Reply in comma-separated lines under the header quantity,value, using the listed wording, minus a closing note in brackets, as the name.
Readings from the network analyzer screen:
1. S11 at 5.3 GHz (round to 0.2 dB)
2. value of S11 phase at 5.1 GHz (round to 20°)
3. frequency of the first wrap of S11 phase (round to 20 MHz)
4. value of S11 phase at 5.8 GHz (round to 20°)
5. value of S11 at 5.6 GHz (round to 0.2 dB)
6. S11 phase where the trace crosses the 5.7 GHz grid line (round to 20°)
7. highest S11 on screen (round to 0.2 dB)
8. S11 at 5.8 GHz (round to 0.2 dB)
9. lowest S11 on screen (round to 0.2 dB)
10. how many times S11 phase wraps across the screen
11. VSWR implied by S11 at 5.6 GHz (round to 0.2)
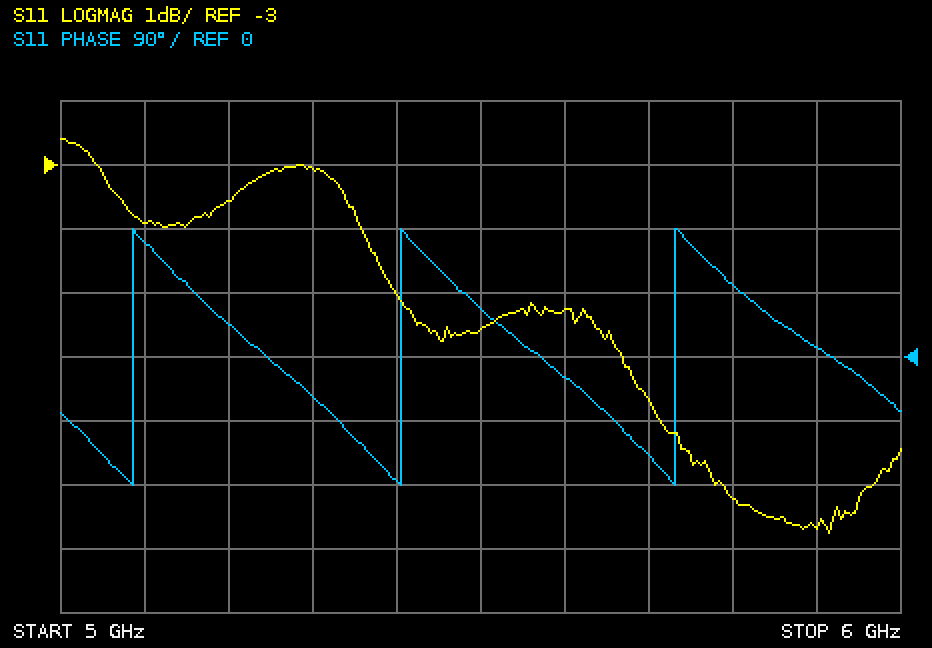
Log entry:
quantity,value
S11 at 5.3 GHz,-3.0 dB
value of S11 phase at 5.1 GHz,160°
frequency of the first wrap of S11 phase,5.08 GHz
value of S11 phase at 5.8 GHz,100°
value of S11 at 5.6 GHz,-5.2 dB
S11 phase where the trace crosses the 5.7 GHz grid line,-140°
highest S11 on screen,-2.6 dB
S11 at 5.8 GHz,-8.2 dB
lowest S11 on screen,-8.8 dB
how many times S11 phase wraps across the screen,3
VSWR implied by S11 at 5.6 GHz,3.4
